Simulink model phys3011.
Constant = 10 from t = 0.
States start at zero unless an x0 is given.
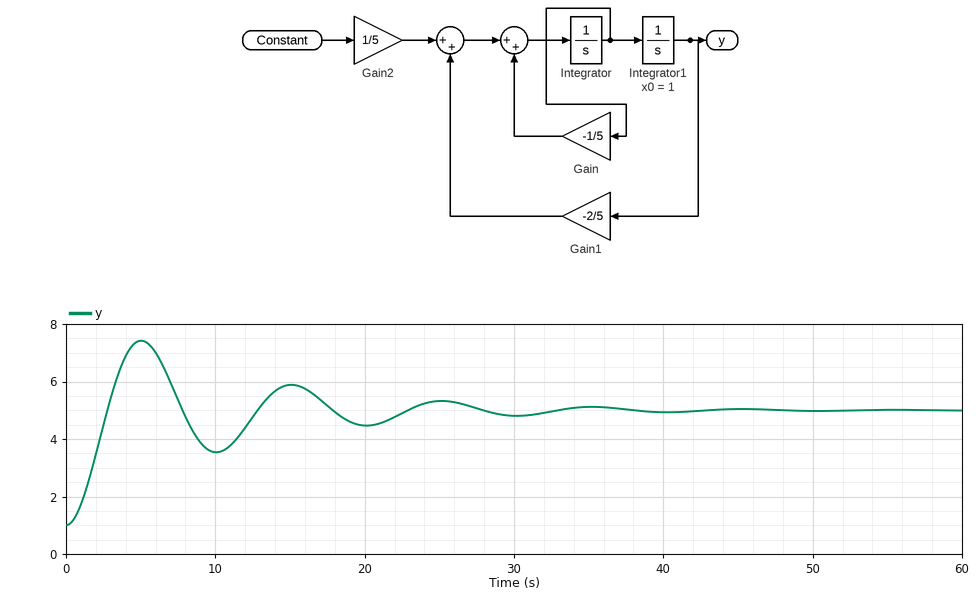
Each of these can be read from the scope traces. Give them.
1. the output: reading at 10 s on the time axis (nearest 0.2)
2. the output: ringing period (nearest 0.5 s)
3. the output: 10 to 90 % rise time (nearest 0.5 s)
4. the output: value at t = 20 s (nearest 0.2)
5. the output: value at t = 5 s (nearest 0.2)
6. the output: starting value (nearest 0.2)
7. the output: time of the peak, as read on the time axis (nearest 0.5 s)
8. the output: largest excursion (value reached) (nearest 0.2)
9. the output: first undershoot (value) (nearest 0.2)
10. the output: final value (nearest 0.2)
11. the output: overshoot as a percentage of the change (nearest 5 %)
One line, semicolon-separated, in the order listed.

3.6; 10.0 s; 2.0 s; 4.4; 7.4; 1.0; 5.0 s; 7.4; 3.6; 5.0; 60 %
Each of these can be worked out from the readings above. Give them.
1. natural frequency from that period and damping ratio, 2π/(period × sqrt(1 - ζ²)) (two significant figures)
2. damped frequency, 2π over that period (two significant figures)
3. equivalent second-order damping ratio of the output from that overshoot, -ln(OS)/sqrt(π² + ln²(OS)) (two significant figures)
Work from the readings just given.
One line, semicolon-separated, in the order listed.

0.64 rad/s; 0.63 rad/s; 0.16
